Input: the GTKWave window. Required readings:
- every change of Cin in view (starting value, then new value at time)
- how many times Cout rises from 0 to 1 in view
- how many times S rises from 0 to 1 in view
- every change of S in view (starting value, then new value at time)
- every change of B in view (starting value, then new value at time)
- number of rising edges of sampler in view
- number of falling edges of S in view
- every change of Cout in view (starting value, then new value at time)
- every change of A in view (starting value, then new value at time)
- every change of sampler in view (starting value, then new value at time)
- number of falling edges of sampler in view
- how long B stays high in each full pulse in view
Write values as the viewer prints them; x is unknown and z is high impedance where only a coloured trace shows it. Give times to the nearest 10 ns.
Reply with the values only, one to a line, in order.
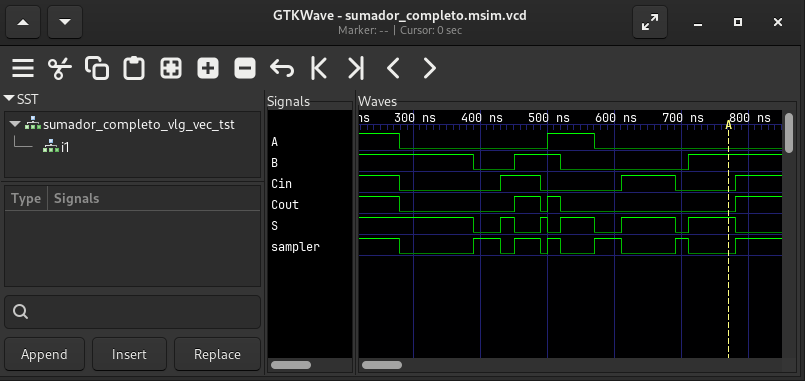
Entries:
1, 0 at 280 ns, 1 at 430 ns, 0 at 490 ns, 1 at 610 ns, 0 at 690 ns, 1 at 780 ns
3
5
1, 0 at 390 ns, 1 at 430 ns, 0 at 450 ns, 1 at 490 ns, 0 at 500 ns, 1 at 520 ns, 0 at 570 ns, 1 at 610 ns, 0 at 690 ns, 1 at 710 ns, 0 at 780 ns
1, 0 at 390 ns, 1 at 450 ns, 0 at 520 ns, 1 at 710 ns
6
6
1, 0 at 280 ns, 1 at 450 ns, 0 at 490 ns, 1 at 500 ns, 0 at 520 ns, 1 at 780 ns
1, 0 at 280 ns, 1 at 500 ns, 0 at 570 ns
1, 0 at 280 ns, 1 at 390 ns, 0 at 430 ns, 1 at 450 ns, 0 at 490 ns, 1 at 500 ns, 0 at 520 ns, 1 at 570 ns, 0 at 610 ns, 1 at 690 ns, 0 at 710 ns, 1 at 780 ns
6
70 ns
